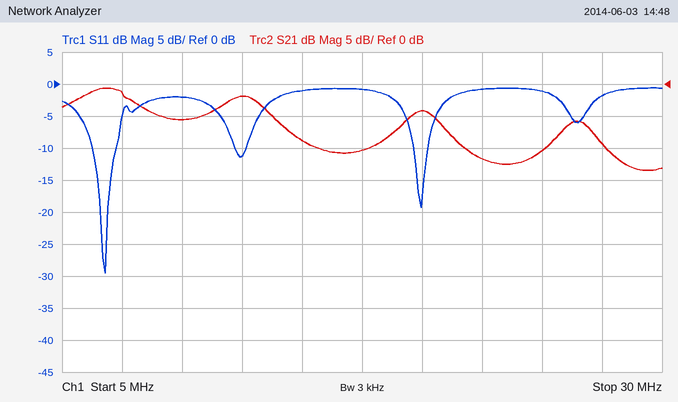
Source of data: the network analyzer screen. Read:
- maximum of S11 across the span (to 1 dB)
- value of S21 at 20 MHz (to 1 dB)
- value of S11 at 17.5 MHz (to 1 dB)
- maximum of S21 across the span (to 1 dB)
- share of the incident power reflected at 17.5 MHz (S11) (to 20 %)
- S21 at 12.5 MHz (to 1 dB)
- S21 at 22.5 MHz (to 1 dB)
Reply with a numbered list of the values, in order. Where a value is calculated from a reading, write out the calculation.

1. -1 dB
2. -4 dB
3. -1 dB
4. -1 dB
5. 10^(-1/10) ≈ 79.4 %, so 80 % to the nearest 20 %
6. -2 dB
7. -12 dB
